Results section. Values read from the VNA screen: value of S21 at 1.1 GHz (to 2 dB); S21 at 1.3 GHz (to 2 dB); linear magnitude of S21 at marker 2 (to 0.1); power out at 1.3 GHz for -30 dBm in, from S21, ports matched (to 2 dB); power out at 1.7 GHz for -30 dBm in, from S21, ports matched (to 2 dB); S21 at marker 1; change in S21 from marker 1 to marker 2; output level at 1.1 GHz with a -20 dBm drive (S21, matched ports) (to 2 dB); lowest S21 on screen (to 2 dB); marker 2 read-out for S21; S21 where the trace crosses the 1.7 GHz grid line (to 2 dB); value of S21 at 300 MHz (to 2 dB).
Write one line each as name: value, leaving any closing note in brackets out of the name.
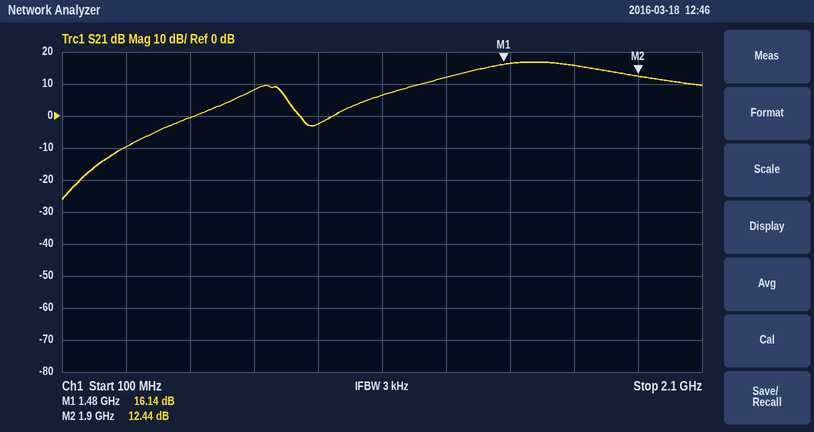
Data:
value of S21 at 1.1 GHz: 6 dB
S21 at 1.3 GHz: 12 dB
linear magnitude of S21 at marker 2: 4.2
power out at 1.3 GHz for -30 dBm in, from S21, ports matched: -18 dBm
power out at 1.7 GHz for -30 dBm in, from S21, ports matched: -14 dBm
S21 at marker 1: 16.14 dB
change in S21 from marker 1 to marker 2: -3.70 dB
output level at 1.1 GHz with a -20 dBm drive (S21, matched ports): -14 dBm
lowest S21 on screen: -26 dB
marker 2 read-out for S21: 12.44 dB
S21 where the trace crosses the 1.7 GHz grid line: 16 dB
value of S21 at 300 MHz: -10 dB
